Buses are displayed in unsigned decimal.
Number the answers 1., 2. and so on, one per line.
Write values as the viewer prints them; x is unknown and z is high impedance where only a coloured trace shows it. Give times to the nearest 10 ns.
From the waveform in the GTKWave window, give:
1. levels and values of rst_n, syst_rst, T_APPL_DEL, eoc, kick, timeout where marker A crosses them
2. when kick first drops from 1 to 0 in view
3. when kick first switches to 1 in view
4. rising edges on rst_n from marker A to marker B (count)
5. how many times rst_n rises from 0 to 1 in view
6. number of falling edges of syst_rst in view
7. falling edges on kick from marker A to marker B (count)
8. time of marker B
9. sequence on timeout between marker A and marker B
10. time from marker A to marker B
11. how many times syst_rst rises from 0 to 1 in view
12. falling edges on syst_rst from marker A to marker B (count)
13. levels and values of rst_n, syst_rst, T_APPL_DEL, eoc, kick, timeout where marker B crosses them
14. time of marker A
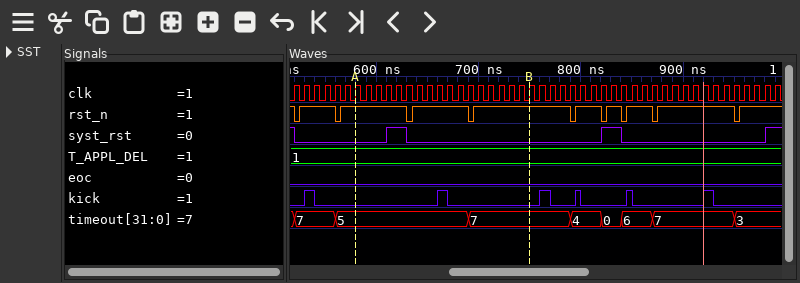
1. rst_n=1, syst_rst=0, T_APPL_DEL=1, eoc=0, kick=0, timeout=5
2. 540 ns
3. 530 ns
4. 2
5. 9
6. 3
7. 1
8. 750 ns
9. 5, 7
10. 170 ns
11. 3
12. 1
13. rst_n=1, syst_rst=0, T_APPL_DEL=1, eoc=0, kick=0, timeout=7
14. 580 ns
